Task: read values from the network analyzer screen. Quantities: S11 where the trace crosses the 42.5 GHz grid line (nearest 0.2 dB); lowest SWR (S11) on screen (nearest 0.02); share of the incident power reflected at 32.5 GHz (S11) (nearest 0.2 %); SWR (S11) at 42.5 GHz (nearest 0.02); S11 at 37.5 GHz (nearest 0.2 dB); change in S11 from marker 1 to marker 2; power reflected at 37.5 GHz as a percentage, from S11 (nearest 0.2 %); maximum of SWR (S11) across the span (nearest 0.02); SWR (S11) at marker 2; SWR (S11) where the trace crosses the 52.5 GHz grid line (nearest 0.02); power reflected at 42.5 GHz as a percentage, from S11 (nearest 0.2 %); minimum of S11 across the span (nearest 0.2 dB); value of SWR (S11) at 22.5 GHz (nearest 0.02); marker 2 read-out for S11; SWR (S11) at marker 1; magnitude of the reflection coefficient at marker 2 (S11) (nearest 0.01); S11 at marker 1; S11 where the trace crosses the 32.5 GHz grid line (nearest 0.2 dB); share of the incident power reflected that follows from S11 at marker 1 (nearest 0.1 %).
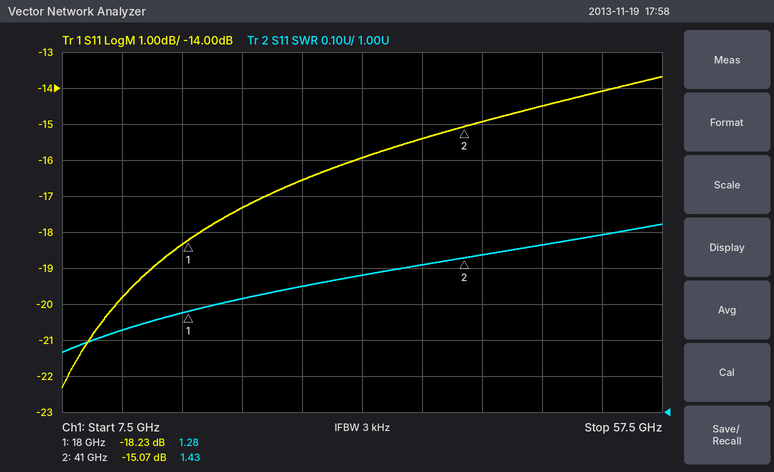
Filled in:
-15.0 dB
1.16
2.6 %
1.44
-15.4 dB
3.16 dB
2.8 %
1.52
1.43
1.50
3.2 %
-22.4 dB
1.32
-15.07 dB
1.28
0.18
-18.23 dB
-16.0 dB
1.5 %
